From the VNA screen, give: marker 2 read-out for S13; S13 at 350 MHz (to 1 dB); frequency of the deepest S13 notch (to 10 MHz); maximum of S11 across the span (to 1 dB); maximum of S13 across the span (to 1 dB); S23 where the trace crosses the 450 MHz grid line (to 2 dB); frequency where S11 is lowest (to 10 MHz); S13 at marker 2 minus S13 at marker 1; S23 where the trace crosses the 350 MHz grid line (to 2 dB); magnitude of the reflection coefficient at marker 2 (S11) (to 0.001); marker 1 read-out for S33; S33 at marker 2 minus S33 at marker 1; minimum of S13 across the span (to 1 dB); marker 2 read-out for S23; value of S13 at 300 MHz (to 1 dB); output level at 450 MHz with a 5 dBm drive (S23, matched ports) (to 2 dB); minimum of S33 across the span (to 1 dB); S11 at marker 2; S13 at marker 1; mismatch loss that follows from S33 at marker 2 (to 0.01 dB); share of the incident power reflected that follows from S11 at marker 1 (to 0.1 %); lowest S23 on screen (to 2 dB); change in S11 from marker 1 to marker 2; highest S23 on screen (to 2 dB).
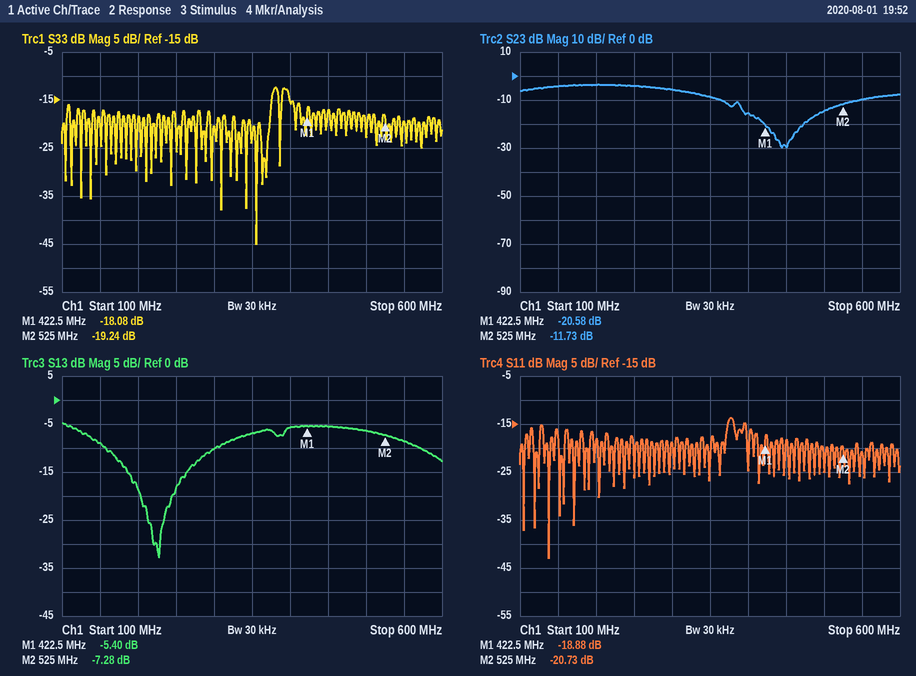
-7.28 dB
-7 dB
230 MHz
-14 dB
-5 dB
-30 dB
140 MHz
-1.88 dB
-8 dB
0.092
-18.08 dB
-1.16 dB
-33 dB
-11.73 dB
-10 dB
-24 dBm
-45 dB
-20.73 dB
-5.40 dB
0.05 dB
1.3 %
-30 dB
-1.85 dB
-4 dB
